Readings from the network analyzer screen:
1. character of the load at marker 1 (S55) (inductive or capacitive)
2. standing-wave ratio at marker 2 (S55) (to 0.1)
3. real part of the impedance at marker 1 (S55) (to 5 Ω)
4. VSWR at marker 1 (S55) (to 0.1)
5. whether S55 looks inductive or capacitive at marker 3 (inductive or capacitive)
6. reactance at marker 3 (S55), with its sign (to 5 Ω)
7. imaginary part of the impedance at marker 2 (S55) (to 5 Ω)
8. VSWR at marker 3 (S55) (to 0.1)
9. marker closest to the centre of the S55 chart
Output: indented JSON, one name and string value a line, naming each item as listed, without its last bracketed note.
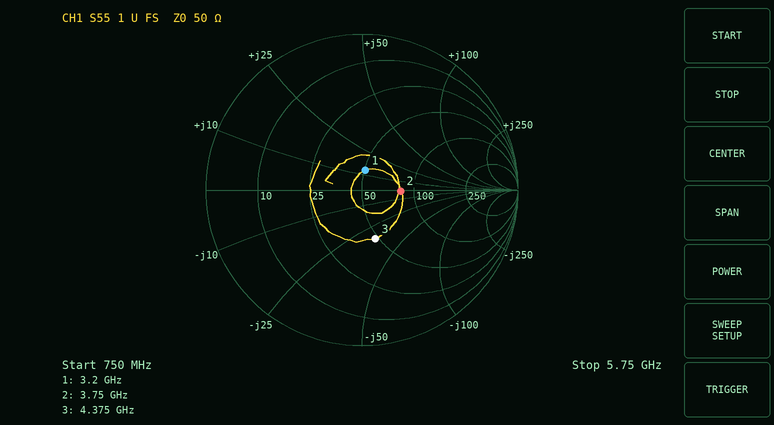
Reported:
{
  "character of the load at marker 1 (S55)": "inductive",
  "standing-wave ratio at marker 2 (S55)": "1.7",
  "real part of the impedance at marker 1 (S55)": "50 Ω",
  "VSWR at marker 1 (S55)": "1.3",
  "whether S55 looks inductive or capacitive at marker 3": "capacitive",
  "reactance at marker 3 (S55), with its sign": "-35 Ω",
  "imaginary part of the impedance at marker 2 (S55)": "0 Ω",
  "VSWR at marker 3 (S55)": "2.0",
  "marker closest to the centre of the S55 chart": "marker 1"
}
